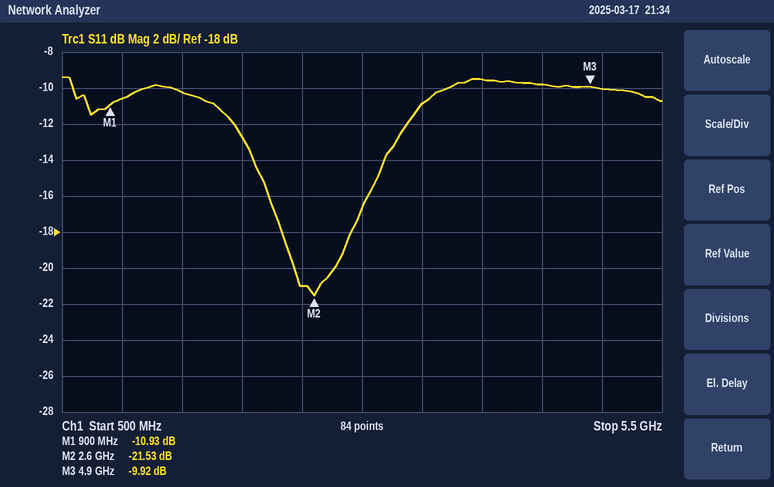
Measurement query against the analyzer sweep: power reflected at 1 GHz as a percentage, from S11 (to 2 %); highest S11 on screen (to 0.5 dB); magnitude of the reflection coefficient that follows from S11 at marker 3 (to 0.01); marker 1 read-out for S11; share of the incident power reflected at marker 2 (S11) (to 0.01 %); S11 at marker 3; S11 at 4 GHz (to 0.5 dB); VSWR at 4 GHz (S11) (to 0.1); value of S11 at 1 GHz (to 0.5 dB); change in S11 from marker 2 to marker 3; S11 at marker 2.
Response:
8 %
-9.5 dB
0.32
-10.93 dB
0.70 %
-9.92 dB
-9.5 dB
2.0
-10.5 dB
11.61 dB
-21.53 dB
